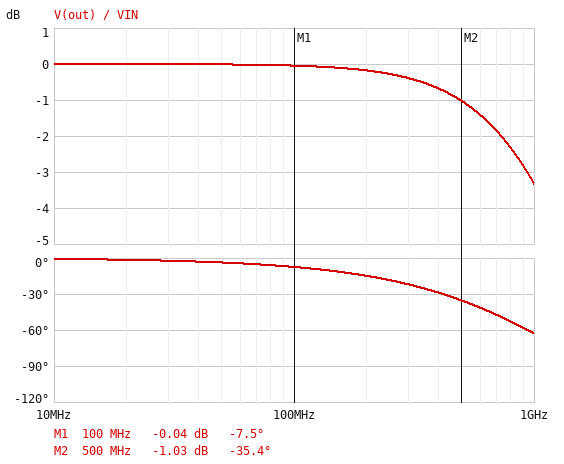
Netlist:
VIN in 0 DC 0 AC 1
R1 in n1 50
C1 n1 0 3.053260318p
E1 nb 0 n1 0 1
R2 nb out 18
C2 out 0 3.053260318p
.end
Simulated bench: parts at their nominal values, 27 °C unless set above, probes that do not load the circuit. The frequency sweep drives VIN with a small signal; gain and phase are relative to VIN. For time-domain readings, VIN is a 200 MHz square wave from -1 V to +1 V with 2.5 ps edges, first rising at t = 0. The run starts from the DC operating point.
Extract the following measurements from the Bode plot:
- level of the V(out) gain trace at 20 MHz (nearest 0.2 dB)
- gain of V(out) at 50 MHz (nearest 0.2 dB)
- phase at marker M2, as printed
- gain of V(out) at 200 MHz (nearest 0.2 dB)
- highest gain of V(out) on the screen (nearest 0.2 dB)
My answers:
0 dB
0 dB
-35.4 deg
-0.2 dB
0 dB
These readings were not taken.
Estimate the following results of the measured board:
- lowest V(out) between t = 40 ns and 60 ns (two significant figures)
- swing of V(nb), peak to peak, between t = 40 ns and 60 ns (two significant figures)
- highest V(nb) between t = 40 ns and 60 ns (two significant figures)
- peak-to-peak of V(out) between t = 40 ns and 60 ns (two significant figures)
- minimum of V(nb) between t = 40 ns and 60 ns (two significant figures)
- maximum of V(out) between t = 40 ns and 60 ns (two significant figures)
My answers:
-1.0 V
2.0 V
1.0 V
2.0 V
-1.0 V
1.0 V
